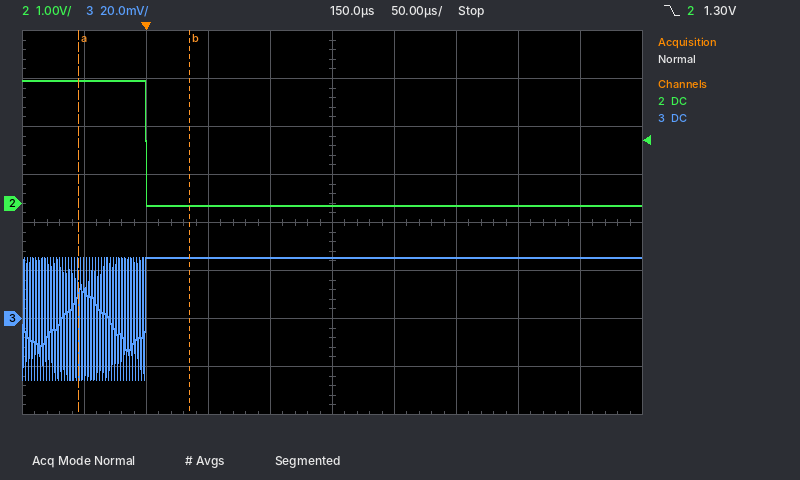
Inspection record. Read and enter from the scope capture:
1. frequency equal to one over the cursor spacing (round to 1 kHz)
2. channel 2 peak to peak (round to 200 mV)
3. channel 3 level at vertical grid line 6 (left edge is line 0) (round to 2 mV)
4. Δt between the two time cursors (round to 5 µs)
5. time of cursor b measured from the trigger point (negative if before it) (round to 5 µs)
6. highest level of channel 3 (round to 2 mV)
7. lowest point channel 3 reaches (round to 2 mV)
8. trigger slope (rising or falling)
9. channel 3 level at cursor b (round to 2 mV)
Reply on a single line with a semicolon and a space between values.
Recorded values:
11 kHz; 2.6 V; 26 mV; 90 µs; +35 µs; 26 mV; -26 mV; falling; 26 mV
